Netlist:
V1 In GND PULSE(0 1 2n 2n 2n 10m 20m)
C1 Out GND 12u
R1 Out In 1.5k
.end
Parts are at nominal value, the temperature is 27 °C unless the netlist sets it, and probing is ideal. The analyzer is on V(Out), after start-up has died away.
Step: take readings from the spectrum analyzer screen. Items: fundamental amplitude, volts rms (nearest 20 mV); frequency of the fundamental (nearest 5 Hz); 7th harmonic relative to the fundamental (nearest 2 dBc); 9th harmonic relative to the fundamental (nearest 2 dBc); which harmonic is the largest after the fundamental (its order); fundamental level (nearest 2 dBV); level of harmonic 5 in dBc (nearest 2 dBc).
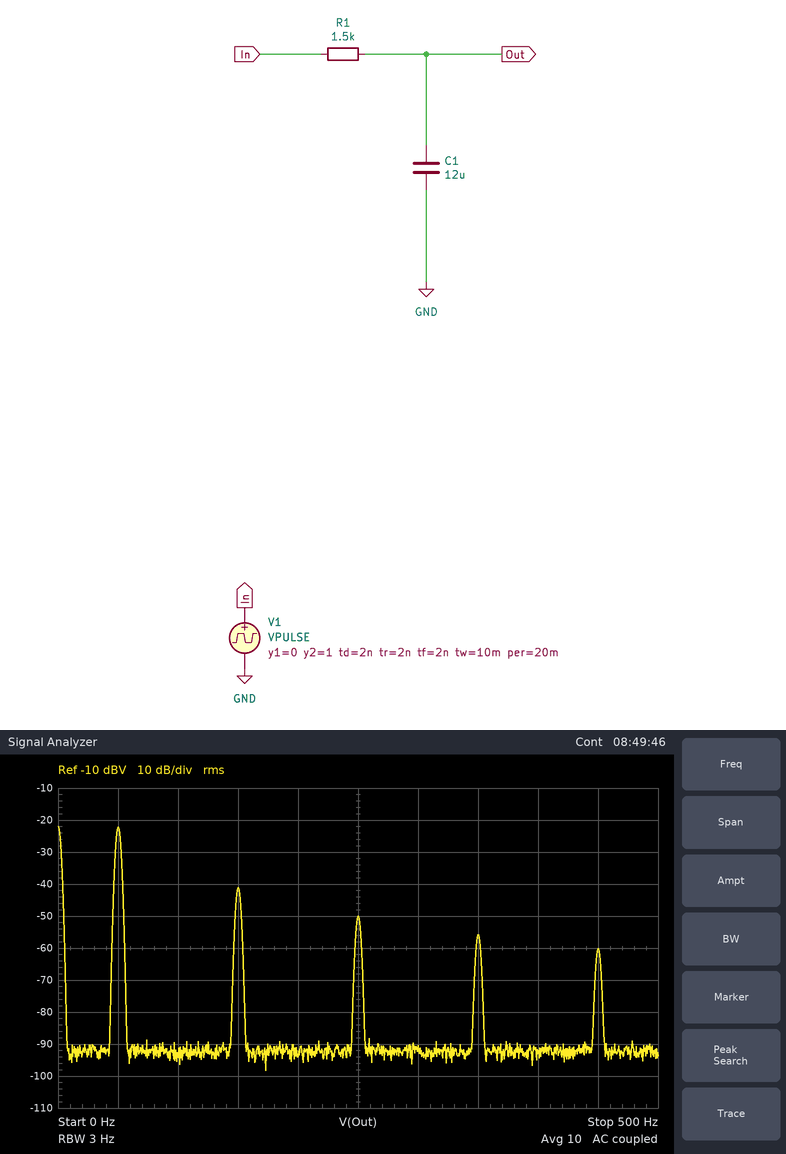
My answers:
80 mV
50 Hz
-34 dBc
-38 dBc
3
-22 dBV
-28 dBc
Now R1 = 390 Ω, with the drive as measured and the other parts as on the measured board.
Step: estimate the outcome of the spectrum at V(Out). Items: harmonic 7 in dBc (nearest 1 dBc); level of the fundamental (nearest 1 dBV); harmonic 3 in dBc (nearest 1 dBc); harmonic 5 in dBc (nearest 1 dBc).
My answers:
-32 dBc
-12 dBV
-18 dBc
-26 dBc
